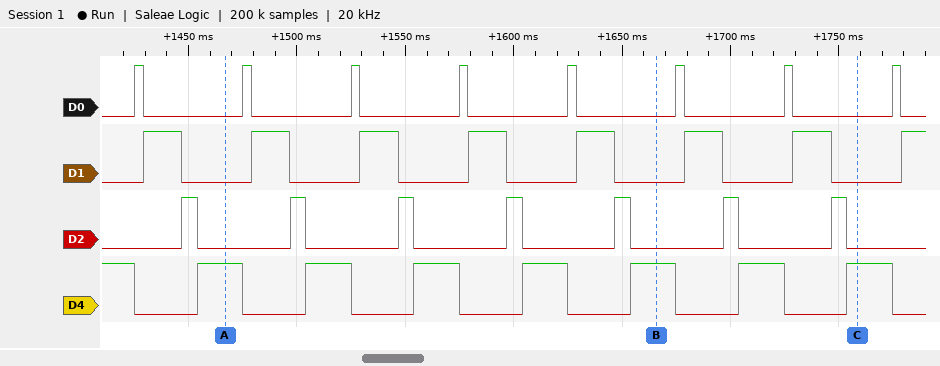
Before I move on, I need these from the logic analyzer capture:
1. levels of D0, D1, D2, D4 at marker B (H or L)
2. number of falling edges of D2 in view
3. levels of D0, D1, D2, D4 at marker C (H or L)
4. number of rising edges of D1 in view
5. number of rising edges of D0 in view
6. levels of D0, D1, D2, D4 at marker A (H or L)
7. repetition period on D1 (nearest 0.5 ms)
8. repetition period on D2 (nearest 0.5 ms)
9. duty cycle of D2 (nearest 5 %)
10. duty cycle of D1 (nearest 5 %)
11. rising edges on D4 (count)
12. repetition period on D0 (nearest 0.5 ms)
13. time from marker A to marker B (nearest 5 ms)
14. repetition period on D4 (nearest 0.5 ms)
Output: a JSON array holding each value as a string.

["D0=L, D1=L, D2=L, D4=H", "7", "D0=L, D1=L, D2=L, D4=H", "8", "8", "D0=L, D1=L, D2=L, D4=H", "50 ms", "50 ms", "15 %", "35 %", "7", "50 ms", "200 ms", "50 ms"]
